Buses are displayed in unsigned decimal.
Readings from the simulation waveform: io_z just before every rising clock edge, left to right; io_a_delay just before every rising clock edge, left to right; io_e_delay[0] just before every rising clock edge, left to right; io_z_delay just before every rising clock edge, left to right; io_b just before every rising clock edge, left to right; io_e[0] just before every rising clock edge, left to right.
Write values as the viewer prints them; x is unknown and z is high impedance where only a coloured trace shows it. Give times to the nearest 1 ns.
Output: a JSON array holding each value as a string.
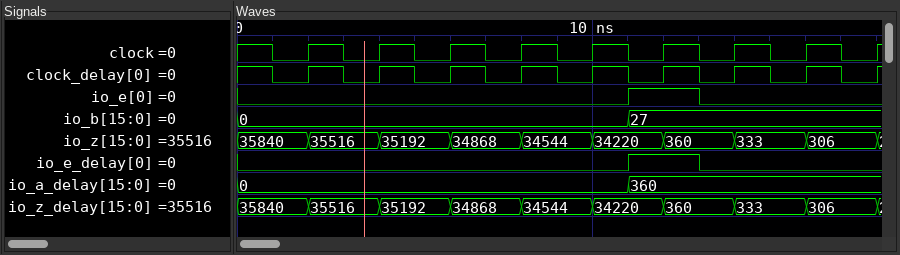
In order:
["35840, 35516, 35192, 34868, 34544, 34220, 360, 333, 306", "0, 0, 0, 0, 0, 360, 360, 360, 360", "0 0 0 0 0 1 0 0 0", "35840, 35516, 35192, 34868, 34544, 34220, 360, 333, 306", "0, 0, 0, 0, 0, 27, 27, 27, 27", "0 0 0 0 0 1 0 0 0"]
